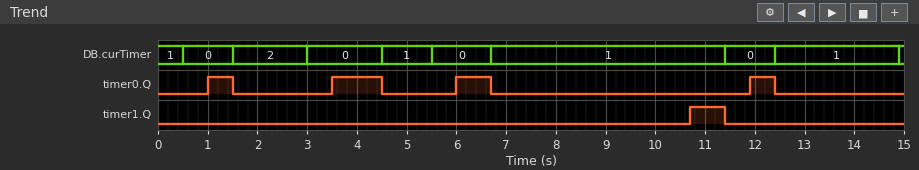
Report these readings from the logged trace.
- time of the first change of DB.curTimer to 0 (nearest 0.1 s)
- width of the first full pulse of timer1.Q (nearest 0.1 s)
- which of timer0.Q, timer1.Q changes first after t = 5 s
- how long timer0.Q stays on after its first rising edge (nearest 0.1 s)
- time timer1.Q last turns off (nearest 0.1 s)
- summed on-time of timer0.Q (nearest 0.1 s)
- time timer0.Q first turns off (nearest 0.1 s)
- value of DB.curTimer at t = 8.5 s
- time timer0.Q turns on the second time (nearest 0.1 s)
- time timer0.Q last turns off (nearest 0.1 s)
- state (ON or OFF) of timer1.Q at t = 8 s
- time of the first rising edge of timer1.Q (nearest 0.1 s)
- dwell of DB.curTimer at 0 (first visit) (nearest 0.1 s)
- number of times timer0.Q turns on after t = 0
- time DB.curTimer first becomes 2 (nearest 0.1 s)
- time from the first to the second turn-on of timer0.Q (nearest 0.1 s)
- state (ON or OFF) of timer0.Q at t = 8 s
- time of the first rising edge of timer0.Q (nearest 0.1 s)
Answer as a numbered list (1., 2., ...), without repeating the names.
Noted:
1. 0.5 s
2. 0.7 s
3. timer0.Q
4. 0.5 s
5. 11.4 s
6. 2.7 s
7. 1.5 s
8. 1
9. 3.5 s
10. 12.4 s
11. OFF
12. 10.7 s
13. 1.0 s
14. 4
15. 1.5 s
16. 2.5 s
17. OFF
18. 1.0 s
